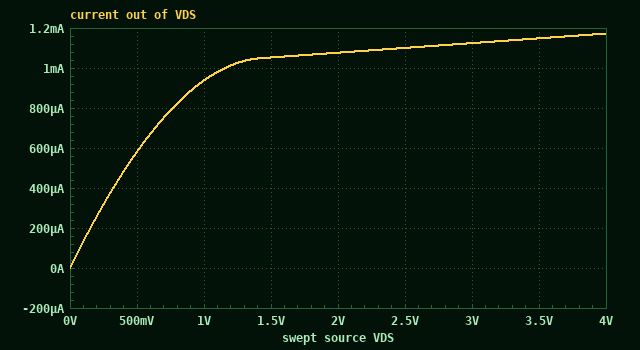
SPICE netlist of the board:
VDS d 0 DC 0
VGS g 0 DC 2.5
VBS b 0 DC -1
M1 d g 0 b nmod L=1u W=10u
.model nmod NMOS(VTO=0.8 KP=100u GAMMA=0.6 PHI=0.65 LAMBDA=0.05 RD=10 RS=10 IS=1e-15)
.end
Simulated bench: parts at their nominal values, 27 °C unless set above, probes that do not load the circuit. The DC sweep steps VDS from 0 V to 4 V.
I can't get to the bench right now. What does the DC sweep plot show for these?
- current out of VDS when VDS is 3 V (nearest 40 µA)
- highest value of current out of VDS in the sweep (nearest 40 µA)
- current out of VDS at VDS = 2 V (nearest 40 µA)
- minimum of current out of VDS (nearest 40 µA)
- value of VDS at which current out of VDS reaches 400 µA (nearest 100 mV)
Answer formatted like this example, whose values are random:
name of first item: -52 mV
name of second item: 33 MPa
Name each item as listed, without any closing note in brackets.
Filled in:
current out of VDS when VDS is 3 V: 1.12 mA
highest value of current out of VDS in the sweep: 1.16 mA
current out of VDS at VDS = 2 V: 1.08 mA
minimum of current out of VDS: 0 A
value of VDS at which current out of VDS reaches 400 µA: 300 mV
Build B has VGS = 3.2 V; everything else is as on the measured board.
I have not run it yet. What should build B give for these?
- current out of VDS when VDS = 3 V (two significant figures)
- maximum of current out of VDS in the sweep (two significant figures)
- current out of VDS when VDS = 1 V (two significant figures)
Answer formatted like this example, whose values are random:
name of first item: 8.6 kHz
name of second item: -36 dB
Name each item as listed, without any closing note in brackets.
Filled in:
current out of VDS when VDS = 3 V: 2.5 mA
maximum of current out of VDS in the sweep: 2.6 mA
current out of VDS when VDS = 1 V: 1.6 mA
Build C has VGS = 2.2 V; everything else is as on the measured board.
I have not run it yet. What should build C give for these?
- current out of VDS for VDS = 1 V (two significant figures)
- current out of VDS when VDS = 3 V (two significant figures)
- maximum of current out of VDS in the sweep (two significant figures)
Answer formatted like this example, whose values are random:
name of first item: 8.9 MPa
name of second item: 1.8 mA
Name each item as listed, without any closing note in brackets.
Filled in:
current out of VDS for VDS = 1 V: 630 µA
current out of VDS when VDS = 3 V: 700 µA
maximum of current out of VDS in the sweep: 730 µA
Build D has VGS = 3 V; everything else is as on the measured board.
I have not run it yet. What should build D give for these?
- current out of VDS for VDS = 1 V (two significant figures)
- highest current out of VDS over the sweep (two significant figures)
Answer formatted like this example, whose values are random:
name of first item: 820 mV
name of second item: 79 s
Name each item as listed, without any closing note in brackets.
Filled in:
current out of VDS for VDS = 1 V: 1.4 mA
highest current out of VDS over the sweep: 2.1 mA
